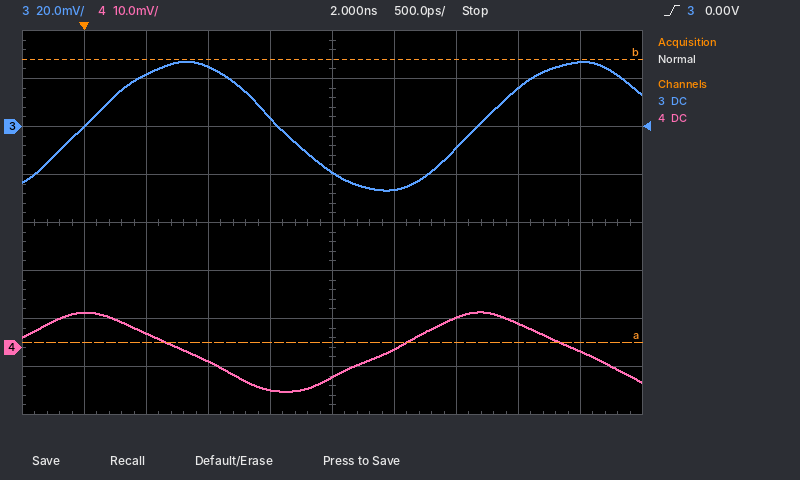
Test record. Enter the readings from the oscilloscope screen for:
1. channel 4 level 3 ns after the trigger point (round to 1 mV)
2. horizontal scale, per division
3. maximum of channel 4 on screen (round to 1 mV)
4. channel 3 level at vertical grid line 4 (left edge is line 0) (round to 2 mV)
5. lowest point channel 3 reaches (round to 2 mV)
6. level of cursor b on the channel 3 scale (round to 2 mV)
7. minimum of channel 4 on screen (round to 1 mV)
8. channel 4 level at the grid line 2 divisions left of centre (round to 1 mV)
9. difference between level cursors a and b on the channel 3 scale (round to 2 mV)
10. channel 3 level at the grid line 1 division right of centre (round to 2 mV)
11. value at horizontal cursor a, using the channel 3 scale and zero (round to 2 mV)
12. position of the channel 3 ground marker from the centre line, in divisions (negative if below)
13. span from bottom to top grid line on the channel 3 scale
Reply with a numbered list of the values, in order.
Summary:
1. 6 mV
2. 500 ps
3. 7 mV
4. 4 mV
5. -26 mV
6. 28 mV
7. -9 mV
8. -3 mV
9. 118 mV
10. -26 mV
11. -90 mV
12. +2.0 div
13. 160 mV
